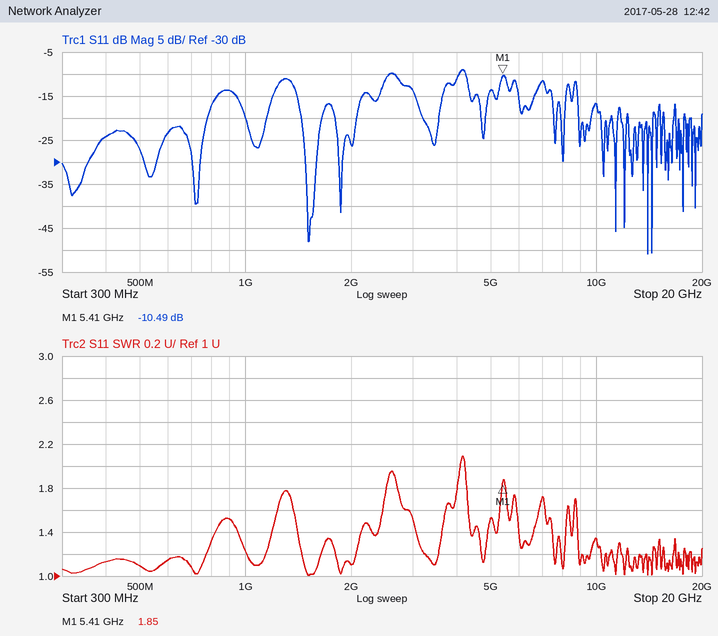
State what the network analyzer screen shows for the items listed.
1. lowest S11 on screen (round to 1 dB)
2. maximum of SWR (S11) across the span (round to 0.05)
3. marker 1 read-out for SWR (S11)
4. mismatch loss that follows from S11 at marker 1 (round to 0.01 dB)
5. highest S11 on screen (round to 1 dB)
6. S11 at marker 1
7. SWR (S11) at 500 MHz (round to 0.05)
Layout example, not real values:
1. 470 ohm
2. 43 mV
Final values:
1. -51 dB
2. 2.10
3. 1.85
4. 0.41 dB
5. -9 dB
6. -10.49 dB
7. 1.10
